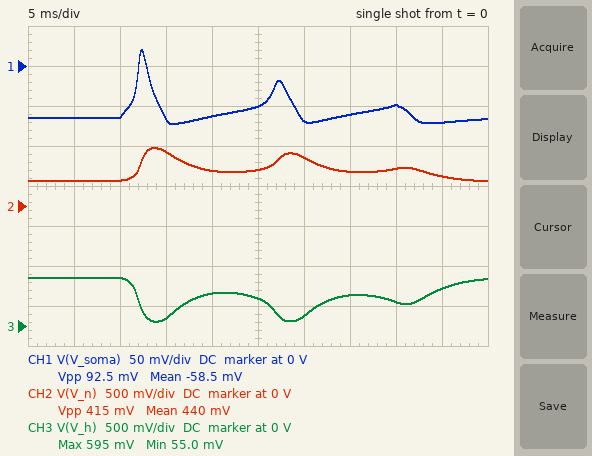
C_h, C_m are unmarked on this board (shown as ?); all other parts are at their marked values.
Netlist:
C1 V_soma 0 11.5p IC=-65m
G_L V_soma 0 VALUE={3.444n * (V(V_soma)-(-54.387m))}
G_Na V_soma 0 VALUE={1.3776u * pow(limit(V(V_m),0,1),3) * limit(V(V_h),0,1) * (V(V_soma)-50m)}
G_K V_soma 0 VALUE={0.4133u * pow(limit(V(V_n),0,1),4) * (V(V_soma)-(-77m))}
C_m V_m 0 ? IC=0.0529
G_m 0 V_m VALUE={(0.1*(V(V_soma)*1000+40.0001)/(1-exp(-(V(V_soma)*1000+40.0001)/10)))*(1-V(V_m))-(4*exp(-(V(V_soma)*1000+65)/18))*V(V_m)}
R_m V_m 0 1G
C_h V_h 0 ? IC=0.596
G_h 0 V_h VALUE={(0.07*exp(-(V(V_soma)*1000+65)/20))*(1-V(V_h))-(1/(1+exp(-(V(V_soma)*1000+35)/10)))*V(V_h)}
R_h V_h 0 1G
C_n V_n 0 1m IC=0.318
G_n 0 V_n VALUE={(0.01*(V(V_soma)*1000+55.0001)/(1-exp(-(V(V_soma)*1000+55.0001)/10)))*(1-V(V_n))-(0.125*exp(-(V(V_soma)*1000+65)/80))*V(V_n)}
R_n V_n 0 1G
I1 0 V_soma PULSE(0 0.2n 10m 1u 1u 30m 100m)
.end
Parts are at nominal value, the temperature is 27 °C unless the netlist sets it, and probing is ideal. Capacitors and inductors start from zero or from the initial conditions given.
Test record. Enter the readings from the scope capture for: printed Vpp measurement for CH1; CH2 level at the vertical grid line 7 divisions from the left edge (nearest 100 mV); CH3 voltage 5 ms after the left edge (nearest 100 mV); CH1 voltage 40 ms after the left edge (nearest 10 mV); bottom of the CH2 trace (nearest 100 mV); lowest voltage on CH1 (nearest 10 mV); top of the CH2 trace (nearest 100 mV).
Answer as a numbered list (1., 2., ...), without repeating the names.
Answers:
1. 92.5 mV
2. 400 mV
3. 600 mV
4. -50 mV
5. 300 mV
6. -70 mV
7. 700 mV
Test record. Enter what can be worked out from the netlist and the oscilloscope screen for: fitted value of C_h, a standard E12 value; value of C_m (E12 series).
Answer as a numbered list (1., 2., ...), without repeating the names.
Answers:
1. 820 µF
2. 2.2 mF
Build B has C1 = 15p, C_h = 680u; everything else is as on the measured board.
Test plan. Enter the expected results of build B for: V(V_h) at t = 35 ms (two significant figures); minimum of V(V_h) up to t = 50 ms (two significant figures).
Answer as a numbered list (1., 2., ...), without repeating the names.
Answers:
1. 400 mV
2. 45 mV
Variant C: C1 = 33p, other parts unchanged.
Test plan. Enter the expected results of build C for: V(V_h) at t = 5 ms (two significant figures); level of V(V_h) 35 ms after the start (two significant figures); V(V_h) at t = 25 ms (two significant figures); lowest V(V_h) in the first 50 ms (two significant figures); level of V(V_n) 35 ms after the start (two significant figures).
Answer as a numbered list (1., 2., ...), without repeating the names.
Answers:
1. 600 mV
2. 110 mV
3. 430 mV
4. 46 mV
5. 600 mV
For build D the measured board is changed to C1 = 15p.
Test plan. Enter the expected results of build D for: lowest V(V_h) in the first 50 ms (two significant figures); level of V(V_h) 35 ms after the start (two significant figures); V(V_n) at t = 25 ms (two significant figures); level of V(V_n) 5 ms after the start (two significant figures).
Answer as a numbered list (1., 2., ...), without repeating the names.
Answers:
1. 53 mV
2. 370 mV
3. 440 mV
4. 320 mV
